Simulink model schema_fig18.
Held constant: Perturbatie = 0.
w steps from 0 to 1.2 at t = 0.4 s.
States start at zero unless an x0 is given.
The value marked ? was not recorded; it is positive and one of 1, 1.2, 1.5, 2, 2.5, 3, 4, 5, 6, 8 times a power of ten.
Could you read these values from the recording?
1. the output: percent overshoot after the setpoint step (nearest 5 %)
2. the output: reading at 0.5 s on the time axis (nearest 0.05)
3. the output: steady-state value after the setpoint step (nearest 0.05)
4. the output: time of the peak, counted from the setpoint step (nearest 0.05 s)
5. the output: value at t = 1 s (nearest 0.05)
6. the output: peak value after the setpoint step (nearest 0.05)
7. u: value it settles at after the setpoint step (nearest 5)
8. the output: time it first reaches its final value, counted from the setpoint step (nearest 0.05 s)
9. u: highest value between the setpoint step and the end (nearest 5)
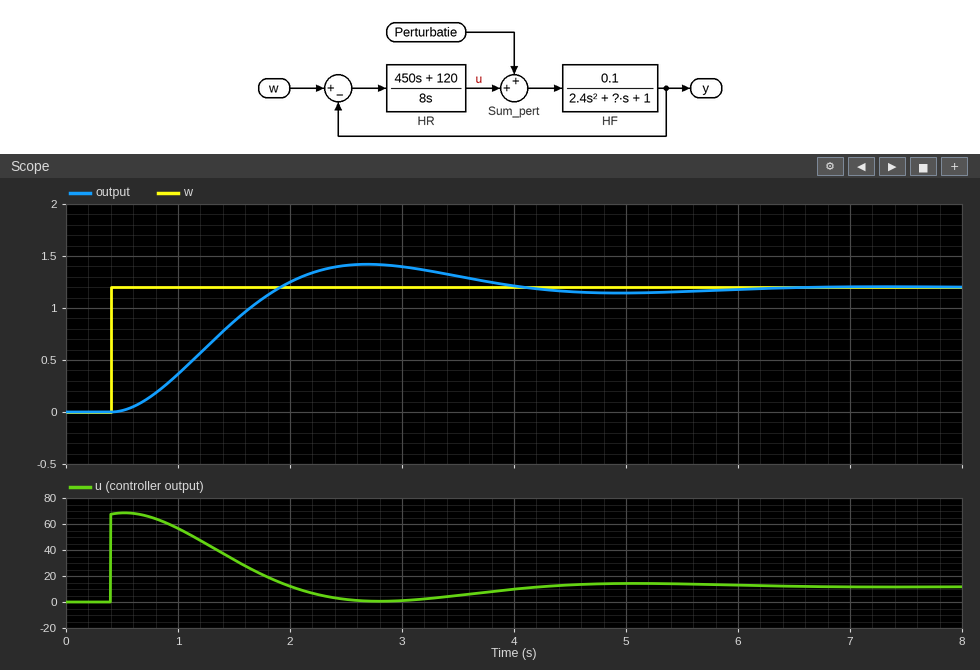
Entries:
20 %
0.00
1.20
2.30 s
0.35
1.40
10
1.50 s
70
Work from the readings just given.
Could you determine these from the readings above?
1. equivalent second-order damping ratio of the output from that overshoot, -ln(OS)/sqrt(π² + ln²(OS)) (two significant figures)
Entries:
0.46
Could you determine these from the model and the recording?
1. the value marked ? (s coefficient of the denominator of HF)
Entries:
4
